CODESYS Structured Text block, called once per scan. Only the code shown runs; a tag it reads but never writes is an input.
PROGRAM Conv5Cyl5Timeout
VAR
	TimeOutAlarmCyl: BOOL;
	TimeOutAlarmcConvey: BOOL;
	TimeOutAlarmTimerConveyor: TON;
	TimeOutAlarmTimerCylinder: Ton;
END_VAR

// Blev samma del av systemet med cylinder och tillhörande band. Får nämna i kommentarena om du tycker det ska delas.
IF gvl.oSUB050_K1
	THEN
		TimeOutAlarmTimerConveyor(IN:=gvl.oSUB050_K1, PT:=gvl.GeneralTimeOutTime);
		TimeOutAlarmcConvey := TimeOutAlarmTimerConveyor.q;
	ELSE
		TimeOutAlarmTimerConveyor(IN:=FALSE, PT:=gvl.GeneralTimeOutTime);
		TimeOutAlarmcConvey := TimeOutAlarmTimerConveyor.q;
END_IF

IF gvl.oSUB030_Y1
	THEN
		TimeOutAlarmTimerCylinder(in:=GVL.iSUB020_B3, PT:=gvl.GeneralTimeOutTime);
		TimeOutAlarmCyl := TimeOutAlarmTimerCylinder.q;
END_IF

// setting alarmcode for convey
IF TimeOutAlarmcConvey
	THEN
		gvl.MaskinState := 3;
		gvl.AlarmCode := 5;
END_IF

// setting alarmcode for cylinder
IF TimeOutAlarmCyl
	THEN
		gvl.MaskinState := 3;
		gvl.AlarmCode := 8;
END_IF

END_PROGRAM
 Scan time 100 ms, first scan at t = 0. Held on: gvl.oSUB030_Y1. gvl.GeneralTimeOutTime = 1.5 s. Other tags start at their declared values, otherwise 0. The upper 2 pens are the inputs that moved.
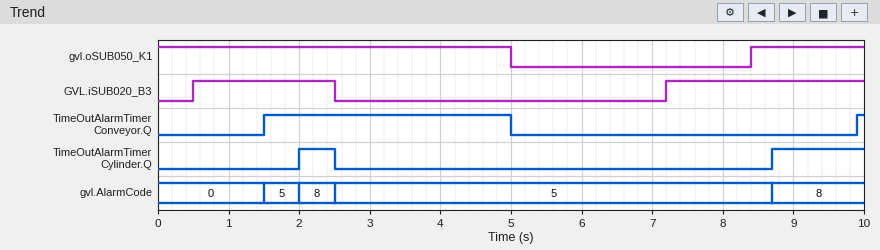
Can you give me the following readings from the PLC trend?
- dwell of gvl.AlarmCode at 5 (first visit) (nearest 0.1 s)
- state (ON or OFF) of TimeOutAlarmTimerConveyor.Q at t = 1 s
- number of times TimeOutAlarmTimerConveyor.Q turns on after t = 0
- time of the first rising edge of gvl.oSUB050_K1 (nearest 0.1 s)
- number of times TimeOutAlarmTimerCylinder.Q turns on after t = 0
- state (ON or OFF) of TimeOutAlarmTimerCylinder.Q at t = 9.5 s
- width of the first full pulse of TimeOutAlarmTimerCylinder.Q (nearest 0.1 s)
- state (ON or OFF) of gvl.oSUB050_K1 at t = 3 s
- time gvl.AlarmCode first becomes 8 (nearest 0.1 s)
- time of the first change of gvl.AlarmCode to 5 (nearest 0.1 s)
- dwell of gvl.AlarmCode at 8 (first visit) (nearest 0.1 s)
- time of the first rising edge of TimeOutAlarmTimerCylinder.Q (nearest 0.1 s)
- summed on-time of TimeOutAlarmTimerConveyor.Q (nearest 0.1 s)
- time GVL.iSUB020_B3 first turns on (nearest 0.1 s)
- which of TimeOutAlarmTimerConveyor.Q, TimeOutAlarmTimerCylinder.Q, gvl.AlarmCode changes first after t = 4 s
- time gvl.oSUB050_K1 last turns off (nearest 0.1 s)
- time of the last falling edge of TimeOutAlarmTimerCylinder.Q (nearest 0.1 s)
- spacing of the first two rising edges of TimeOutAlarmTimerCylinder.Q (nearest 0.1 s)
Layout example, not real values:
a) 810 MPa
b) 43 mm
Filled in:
a) 0.5 s
b) OFF
c) 2
d) 8.4 s
e) 2
f) ON
g) 0.5 s
h) ON
i) 2.0 s
j) 1.5 s
k) 0.5 s
l) 2.0 s
m) 3.6 s
n) 0.5 s
o) TimeOutAlarmTimerConveyor.Q
p) 5.0 s
q) 2.5 s
r) 6.7 s
